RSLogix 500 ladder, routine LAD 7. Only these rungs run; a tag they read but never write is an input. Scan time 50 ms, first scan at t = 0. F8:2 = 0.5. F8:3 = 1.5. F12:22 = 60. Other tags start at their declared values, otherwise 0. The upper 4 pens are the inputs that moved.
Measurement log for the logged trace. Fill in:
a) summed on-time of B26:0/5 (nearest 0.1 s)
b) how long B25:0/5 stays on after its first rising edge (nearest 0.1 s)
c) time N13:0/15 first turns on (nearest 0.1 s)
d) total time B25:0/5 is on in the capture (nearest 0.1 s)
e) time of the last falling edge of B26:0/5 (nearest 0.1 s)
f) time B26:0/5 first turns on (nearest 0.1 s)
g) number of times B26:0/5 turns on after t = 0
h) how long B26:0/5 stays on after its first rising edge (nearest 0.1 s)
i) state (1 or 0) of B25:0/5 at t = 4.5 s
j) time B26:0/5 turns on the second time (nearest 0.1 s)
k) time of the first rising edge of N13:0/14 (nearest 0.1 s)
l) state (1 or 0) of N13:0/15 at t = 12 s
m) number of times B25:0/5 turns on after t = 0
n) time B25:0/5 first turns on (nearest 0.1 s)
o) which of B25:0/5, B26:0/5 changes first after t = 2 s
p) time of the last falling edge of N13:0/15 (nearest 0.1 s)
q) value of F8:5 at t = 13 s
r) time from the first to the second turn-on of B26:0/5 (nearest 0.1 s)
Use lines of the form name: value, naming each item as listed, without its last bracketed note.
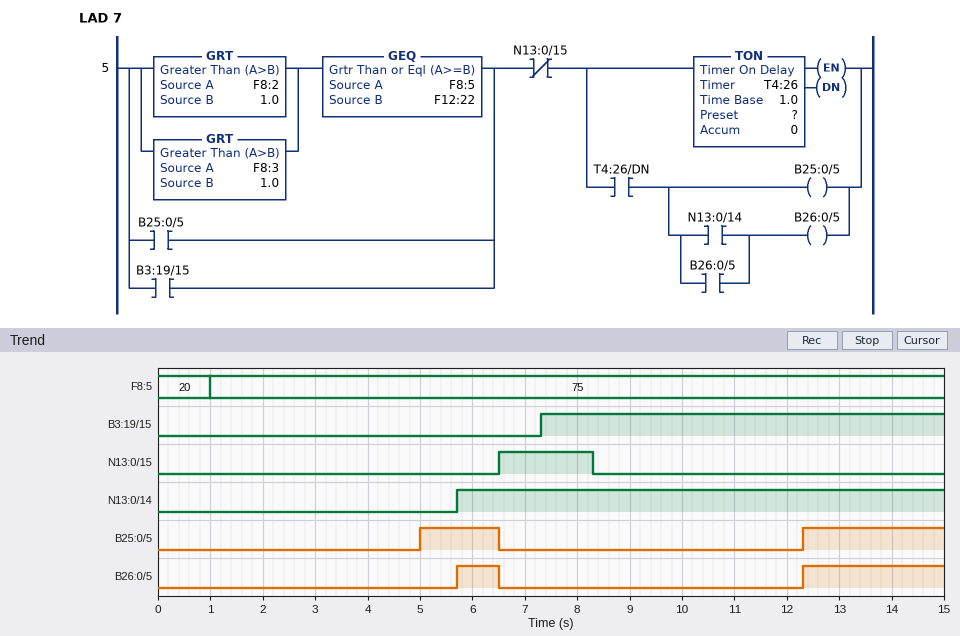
summed on-time of B26:0/5: 3.5 s
how long B25:0/5 stays on after its first rising edge: 1.5 s
time N13:0/15 first turns on: 6.5 s
total time B25:0/5 is on in the capture: 4.2 s
time of the last falling edge of B26:0/5: 6.5 s
time B26:0/5 first turns on: 5.7 s
number of times B26:0/5 turns on after t = 0: 2
how long B26:0/5 stays on after its first rising edge: 0.8 s
state (1 or 0) of B25:0/5 at t = 4.5 s: 0
time B26:0/5 turns on the second time: 12.3 s
time of the first rising edge of N13:0/14: 5.7 s
state (1 or 0) of N13:0/15 at t = 12 s: 0
number of times B25:0/5 turns on after t = 0: 2
time B25:0/5 first turns on: 5.0 s
which of B25:0/5, B26:0/5 changes first after t = 2 s: B25:0/5
time of the last falling edge of N13:0/15: 8.3 s
value of F8:5 at t = 13 s: 75
time from the first to the second turn-on of B26:0/5: 6.6 s
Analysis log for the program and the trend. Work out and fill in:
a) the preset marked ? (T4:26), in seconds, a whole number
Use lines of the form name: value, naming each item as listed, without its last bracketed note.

the preset marked ? (T4:26), in seconds, a whole number: 4 s
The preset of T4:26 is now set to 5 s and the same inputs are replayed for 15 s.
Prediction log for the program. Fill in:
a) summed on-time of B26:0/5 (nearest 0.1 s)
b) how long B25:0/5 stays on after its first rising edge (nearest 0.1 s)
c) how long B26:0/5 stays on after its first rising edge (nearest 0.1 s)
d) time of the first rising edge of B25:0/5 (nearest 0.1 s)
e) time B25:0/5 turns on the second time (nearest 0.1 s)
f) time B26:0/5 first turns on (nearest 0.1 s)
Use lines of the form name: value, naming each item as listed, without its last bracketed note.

summed on-time of B26:0/5: 2.2 s
how long B25:0/5 stays on after its first rising edge: 0.5 s
how long B26:0/5 stays on after its first rising edge: 0.5 s
time of the first rising edge of B25:0/5: 6.0 s
time B25:0/5 turns on the second time: 13.3 s
time B26:0/5 first turns on: 6.0 s
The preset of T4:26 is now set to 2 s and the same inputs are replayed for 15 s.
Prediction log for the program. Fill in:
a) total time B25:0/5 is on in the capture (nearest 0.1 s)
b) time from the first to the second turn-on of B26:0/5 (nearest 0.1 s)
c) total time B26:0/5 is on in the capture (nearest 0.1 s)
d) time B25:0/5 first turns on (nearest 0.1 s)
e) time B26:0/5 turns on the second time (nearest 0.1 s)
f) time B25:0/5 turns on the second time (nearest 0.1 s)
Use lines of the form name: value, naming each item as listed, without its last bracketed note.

total time B25:0/5 is on in the capture: 8.2 s
time from the first to the second turn-on of B26:0/5: 4.6 s
total time B26:0/5 is on in the capture: 5.5 s
time B25:0/5 first turns on: 3.0 s
time B26:0/5 turns on the second time: 10.3 s
time B25:0/5 turns on the second time: 10.3 s
